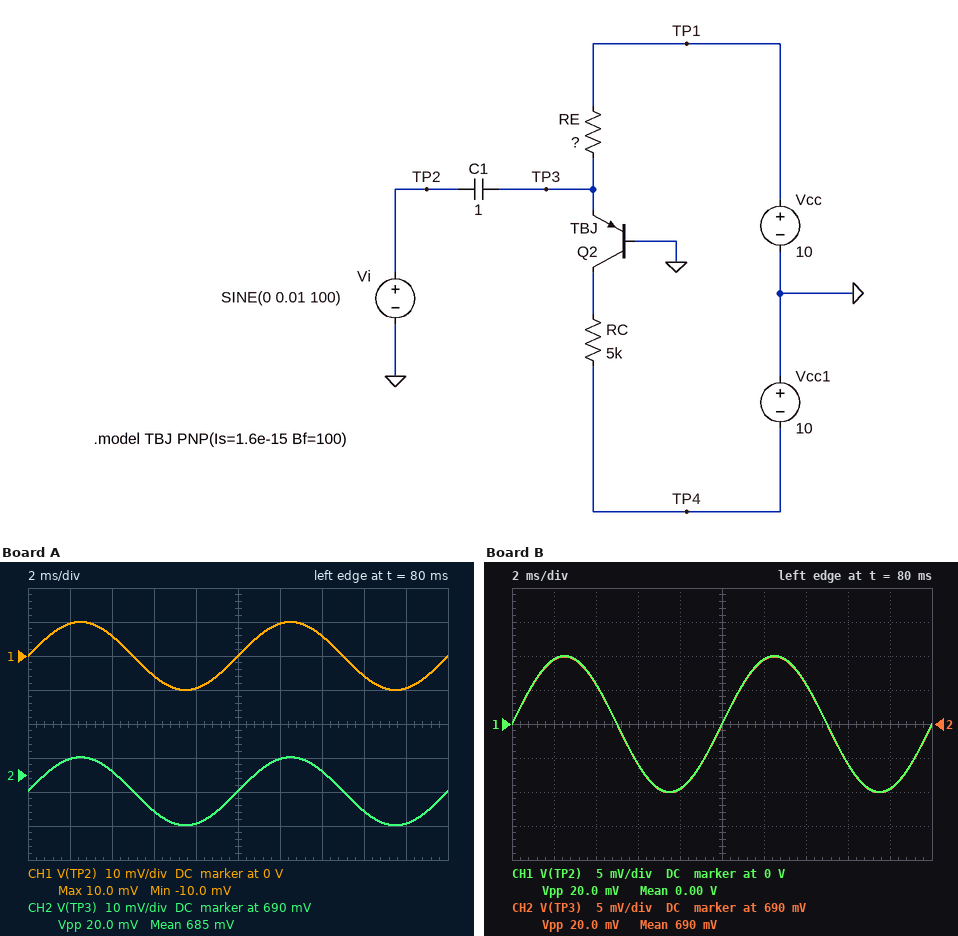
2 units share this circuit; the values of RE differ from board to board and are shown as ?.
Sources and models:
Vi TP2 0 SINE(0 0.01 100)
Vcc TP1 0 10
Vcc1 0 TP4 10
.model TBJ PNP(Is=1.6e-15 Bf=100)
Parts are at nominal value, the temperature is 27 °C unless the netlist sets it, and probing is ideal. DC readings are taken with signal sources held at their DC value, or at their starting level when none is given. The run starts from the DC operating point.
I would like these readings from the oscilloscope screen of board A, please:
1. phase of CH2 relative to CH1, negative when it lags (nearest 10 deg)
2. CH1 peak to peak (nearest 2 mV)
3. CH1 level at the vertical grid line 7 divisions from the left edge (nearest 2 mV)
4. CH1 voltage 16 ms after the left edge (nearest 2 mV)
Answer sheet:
0 deg
20 mV
6 mV
-6 mV
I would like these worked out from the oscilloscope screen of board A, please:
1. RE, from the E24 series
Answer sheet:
18 kΩ
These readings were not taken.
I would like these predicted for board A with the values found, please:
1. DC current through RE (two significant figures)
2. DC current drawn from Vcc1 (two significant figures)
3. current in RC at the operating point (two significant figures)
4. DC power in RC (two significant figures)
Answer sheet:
520 µA
510 µA
510 µA
1.3 mW
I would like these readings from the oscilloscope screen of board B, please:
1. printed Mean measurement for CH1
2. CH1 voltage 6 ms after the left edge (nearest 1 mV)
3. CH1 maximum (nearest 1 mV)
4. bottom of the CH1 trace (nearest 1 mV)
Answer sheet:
0.00 V
-6 mV
10 mV
-10 mV
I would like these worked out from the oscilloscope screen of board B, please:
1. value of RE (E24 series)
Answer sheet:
15 kΩ
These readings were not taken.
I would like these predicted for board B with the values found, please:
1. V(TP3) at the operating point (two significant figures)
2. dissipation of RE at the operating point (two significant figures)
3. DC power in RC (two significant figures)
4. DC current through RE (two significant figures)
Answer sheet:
690 mV
5.8 mW
1.9 mW
620 µA
